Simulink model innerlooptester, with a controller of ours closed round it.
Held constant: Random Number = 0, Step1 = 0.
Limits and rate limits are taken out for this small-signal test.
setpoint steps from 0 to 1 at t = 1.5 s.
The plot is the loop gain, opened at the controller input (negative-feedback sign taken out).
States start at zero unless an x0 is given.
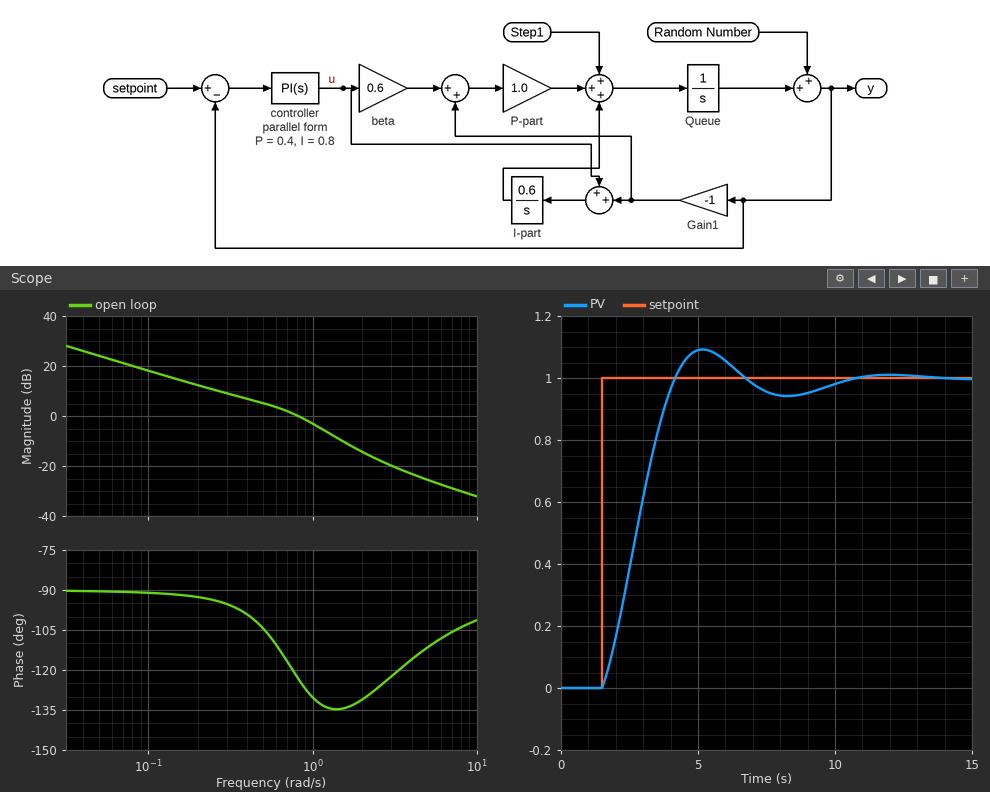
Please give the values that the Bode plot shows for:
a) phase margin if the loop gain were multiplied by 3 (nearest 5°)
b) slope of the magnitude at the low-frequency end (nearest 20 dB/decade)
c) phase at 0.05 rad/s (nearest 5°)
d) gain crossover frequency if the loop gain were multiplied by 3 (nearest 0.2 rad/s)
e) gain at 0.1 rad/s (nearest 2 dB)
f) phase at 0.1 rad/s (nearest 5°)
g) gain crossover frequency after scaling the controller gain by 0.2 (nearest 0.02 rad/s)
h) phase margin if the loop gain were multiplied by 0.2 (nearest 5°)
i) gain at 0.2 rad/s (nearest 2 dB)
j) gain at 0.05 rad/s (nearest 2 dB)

45°
-20 dB/decade
-90°
1.4 rad/s
18 dB
-90°
0.16 rad/s
90°
12 dB
24 dB
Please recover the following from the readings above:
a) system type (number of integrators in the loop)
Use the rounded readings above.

1
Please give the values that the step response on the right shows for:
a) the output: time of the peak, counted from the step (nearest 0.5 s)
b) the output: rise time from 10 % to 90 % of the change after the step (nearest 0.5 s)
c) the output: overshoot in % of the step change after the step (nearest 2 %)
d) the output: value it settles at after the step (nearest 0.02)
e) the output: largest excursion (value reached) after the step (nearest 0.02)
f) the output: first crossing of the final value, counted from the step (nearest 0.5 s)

3.5 s
2.0 s
10 %
1.00
1.10
2.5 s
